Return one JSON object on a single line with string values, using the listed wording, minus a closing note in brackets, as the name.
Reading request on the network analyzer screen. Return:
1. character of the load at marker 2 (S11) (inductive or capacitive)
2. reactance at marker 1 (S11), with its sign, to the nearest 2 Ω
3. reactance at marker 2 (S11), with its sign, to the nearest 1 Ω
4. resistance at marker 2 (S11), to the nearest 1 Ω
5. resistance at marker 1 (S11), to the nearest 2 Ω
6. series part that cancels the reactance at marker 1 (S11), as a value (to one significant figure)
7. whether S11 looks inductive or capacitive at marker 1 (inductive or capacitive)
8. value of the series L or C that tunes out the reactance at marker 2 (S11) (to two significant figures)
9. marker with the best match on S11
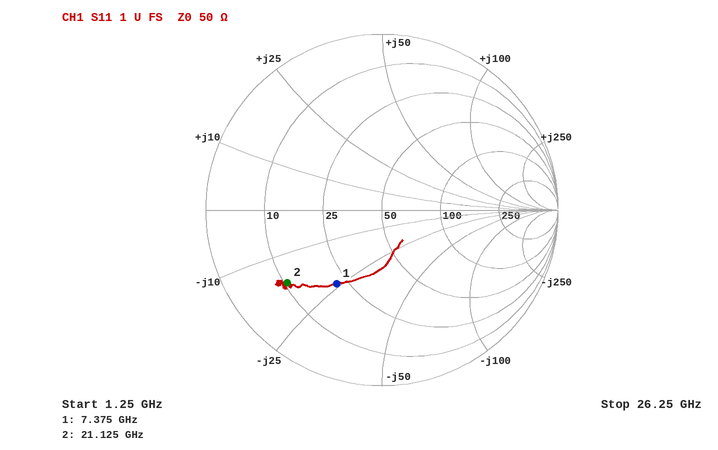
{"character of the load at marker 2 (S11)": "capacitive", "reactance at marker 1 (S11), with its sign, to the nearest 2 Ω": "-24 Ω", "reactance at marker 2 (S11), with its sign, to the nearest 1 Ω": "-16 Ω", "resistance at marker 2 (S11), to the nearest 1 Ω": "11 Ω", "resistance at marker 1 (S11), to the nearest 2 Ω": "22 Ω", "series part that cancels the reactance at marker 1 (S11), as a value": "500 pH", "whether S11 looks inductive or capacitive at marker 1": "capacitive", "value of the series L or C that tunes out the reactance at marker 2 (S11)": "120 pH", "marker with the best match on S11": "marker 1"}
